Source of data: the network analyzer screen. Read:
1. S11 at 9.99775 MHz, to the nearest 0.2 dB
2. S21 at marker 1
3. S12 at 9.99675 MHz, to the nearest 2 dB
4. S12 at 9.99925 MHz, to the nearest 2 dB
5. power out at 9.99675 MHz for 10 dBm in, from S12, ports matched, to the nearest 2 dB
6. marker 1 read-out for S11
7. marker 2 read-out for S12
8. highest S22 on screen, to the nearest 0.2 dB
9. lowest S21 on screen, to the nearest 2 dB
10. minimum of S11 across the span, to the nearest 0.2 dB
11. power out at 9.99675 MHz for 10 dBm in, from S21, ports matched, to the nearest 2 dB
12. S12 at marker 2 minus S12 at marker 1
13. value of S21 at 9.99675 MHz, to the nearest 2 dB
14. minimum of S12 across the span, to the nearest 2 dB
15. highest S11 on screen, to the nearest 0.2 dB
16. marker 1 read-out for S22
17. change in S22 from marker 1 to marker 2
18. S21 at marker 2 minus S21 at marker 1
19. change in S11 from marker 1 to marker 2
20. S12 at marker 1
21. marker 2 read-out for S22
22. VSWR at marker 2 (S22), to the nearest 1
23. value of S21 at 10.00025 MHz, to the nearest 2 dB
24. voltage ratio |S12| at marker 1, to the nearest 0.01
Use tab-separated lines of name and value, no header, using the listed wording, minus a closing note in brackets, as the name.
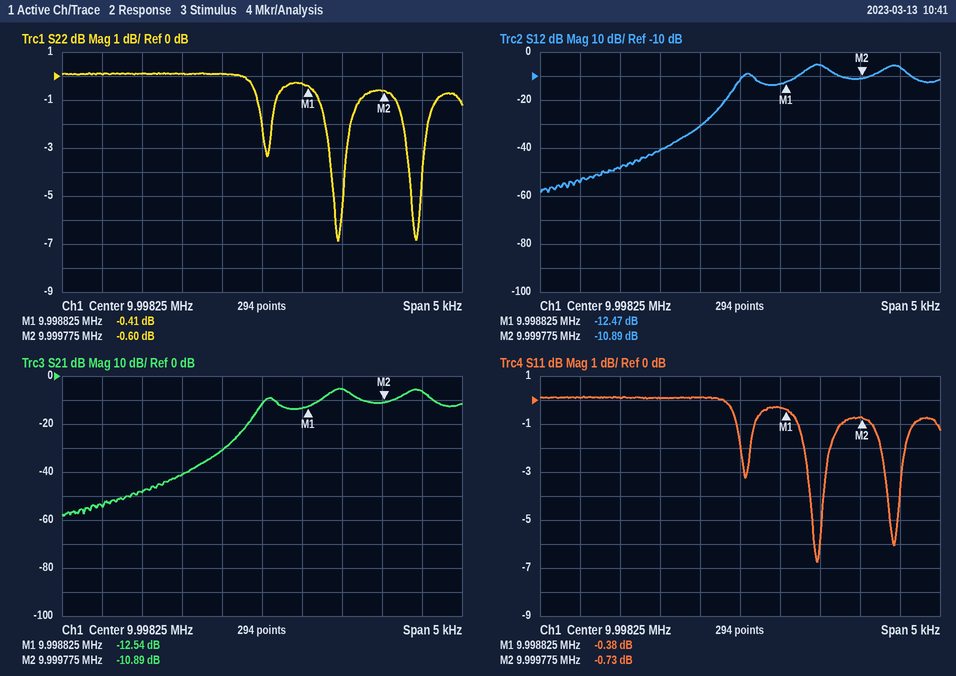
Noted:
S11 at 9.99775 MHz, to the nearest 0.2 dB	0.2 dB
S21 at marker 1	-12.54 dB
S12 at 9.99675 MHz, to the nearest 2 dB	-48 dB
S12 at 9.99925 MHz, to the nearest 2 dB	-6 dB
power out at 9.99675 MHz for 10 dBm in, from S12, ports matched, to the nearest 2 dB	-38 dBm
marker 1 read-out for S11	-0.38 dB
marker 2 read-out for S12	-10.89 dB
highest S22 on screen, to the nearest 0.2 dB	0.2 dB
lowest S21 on screen, to the nearest 2 dB	-58 dB
minimum of S11 across the span, to the nearest 0.2 dB	-6.8 dB
power out at 9.99675 MHz for 10 dBm in, from S21, ports matched, to the nearest 2 dB	-38 dBm
S12 at marker 2 minus S12 at marker 1	1.58 dB
value of S21 at 9.99675 MHz, to the nearest 2 dB	-48 dB
minimum of S12 across the span, to the nearest 2 dB	-58 dB
highest S11 on screen, to the nearest 0.2 dB	0.2 dB
marker 1 read-out for S22	-0.41 dB
change in S22 from marker 1 to marker 2	-0.19 dB
S21 at marker 2 minus S21 at marker 1	1.65 dB
change in S11 from marker 1 to marker 2	-0.35 dB
S12 at marker 1	-12.47 dB
marker 2 read-out for S22	-0.60 dB
VSWR at marker 2 (S22), to the nearest 1	29
value of S21 at 10.00025 MHz, to the nearest 2 dB	-6 dB
voltage ratio |S12| at marker 1, to the nearest 0.01	0.24
